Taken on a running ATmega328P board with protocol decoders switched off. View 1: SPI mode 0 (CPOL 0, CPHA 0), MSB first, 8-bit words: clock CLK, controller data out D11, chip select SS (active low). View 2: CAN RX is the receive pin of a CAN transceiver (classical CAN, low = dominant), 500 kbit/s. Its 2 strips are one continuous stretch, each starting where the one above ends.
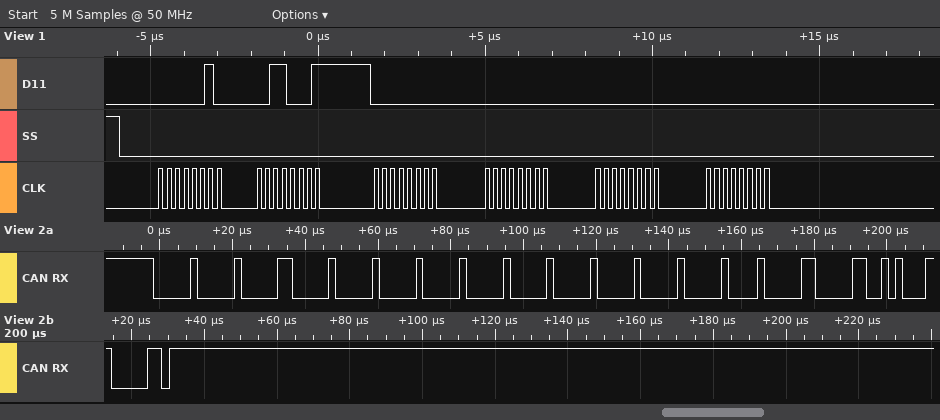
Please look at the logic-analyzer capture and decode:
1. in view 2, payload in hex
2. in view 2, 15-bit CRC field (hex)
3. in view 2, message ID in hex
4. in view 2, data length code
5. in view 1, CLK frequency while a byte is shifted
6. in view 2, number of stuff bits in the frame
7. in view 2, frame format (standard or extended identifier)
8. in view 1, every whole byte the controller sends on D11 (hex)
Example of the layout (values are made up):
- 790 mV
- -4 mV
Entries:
- 00 00 00 00 00 00 10 41
- 0x1460
- 0x000
- 8
- 4 MHz
- 16
- standard
- 02 31 00 00 00 00
